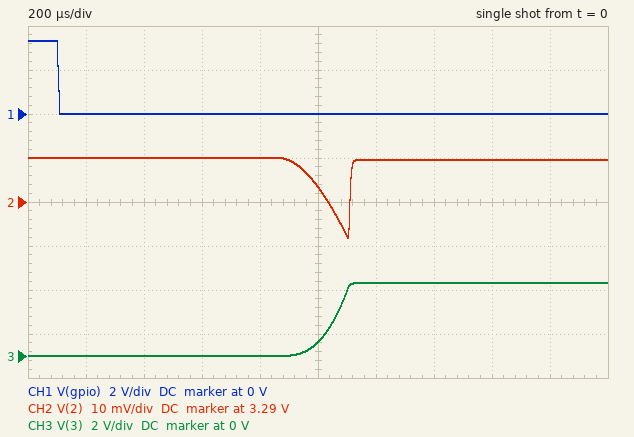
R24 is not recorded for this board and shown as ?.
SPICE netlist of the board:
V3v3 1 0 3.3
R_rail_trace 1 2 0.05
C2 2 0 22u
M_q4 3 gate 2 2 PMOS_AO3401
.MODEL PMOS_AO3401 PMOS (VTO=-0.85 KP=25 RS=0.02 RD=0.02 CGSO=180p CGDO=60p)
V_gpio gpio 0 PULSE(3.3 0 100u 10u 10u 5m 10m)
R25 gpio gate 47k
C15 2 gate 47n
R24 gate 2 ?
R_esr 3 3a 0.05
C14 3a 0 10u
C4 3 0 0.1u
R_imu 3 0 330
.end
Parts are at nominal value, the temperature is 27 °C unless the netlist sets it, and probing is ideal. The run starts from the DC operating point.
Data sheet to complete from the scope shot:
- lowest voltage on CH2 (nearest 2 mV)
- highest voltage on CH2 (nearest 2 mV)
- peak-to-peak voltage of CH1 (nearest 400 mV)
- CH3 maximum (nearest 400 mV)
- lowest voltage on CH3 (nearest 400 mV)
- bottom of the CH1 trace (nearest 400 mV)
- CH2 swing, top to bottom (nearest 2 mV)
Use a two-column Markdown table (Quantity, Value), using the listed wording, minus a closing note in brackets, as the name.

| Quantity | Value |
|---|---|
| lowest voltage on CH2 | 3.282 V |
| highest voltage on CH2 | 3.300 V |
| peak-to-peak voltage of CH1 | 3.2 V |
| CH3 maximum | 3.2 V |
| lowest voltage on CH3 | 0 V |
| bottom of the CH1 trace | 0 V |
| CH2 swing, top to bottom | 18 mV |
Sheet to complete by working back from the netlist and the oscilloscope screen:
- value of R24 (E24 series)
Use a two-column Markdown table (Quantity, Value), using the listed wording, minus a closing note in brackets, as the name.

| Quantity | Value |
|---|---|
| value of R24 | 62 kΩ |
